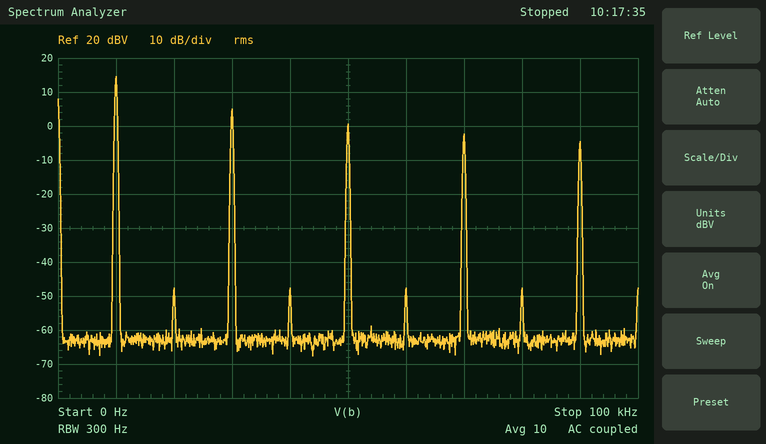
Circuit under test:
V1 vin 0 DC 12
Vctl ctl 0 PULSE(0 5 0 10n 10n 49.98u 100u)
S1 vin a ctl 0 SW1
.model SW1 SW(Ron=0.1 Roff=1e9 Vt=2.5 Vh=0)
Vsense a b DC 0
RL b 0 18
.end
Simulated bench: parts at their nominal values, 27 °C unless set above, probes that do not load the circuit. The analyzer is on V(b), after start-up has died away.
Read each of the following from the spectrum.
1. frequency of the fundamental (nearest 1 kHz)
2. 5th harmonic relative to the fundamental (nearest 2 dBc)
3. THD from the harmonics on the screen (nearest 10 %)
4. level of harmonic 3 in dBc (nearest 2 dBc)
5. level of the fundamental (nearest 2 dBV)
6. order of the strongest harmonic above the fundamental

10 kHz
-14 dBc
40 %
-10 dBc
14 dBV
3
